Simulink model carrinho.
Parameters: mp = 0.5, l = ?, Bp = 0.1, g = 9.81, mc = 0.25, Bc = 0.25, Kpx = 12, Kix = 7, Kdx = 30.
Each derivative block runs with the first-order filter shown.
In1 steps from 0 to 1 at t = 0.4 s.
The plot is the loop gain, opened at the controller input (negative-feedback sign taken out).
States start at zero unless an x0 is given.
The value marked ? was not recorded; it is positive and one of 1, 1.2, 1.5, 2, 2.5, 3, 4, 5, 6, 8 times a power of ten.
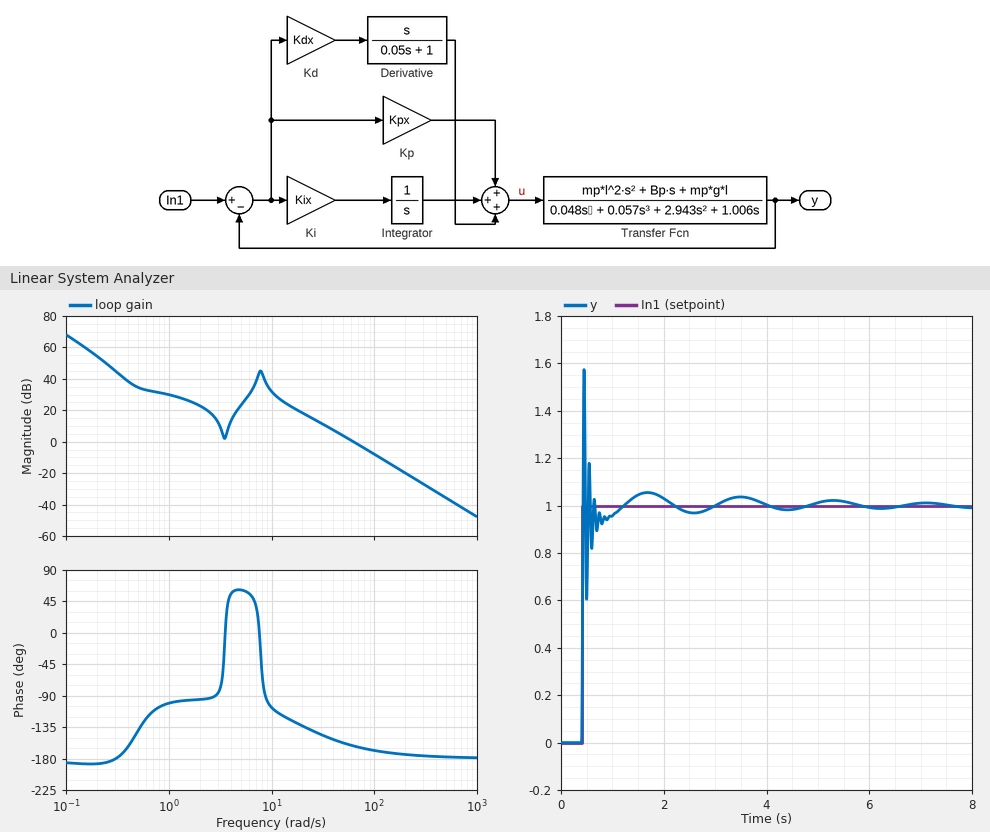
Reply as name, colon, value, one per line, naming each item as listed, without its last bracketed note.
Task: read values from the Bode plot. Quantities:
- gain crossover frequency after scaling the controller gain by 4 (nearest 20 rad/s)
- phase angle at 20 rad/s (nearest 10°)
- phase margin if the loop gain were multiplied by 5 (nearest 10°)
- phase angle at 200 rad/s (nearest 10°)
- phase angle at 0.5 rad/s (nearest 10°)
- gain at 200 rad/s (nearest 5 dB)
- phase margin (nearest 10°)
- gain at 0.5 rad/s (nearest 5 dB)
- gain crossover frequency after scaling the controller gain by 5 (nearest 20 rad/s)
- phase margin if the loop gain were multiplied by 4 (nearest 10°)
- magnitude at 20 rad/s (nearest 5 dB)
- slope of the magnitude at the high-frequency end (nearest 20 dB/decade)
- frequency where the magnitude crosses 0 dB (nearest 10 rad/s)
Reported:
gain crossover frequency after scaling the controller gain by 4: 120 rad/s
phase angle at 20 rad/s: -130°
phase margin if the loop gain were multiplied by 5: 10°
phase angle at 200 rad/s: -170°
phase angle at 0.5 rad/s: -140°
gain at 200 rad/s: -20 dB
phase margin: 20°
gain at 0.5 rad/s: 35 dB
gain crossover frequency after scaling the controller gain by 5: 140 rad/s
phase margin if the loop gain were multiplied by 4: 10°
magnitude at 20 rad/s: 20 dB
slope of the magnitude at the high-frequency end: -40 dB/decade
frequency where the magnitude crosses 0 dB: 60 rad/s
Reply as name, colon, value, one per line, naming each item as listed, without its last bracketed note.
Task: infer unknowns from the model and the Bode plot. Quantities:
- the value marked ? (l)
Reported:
the value marked ?: 0.8
